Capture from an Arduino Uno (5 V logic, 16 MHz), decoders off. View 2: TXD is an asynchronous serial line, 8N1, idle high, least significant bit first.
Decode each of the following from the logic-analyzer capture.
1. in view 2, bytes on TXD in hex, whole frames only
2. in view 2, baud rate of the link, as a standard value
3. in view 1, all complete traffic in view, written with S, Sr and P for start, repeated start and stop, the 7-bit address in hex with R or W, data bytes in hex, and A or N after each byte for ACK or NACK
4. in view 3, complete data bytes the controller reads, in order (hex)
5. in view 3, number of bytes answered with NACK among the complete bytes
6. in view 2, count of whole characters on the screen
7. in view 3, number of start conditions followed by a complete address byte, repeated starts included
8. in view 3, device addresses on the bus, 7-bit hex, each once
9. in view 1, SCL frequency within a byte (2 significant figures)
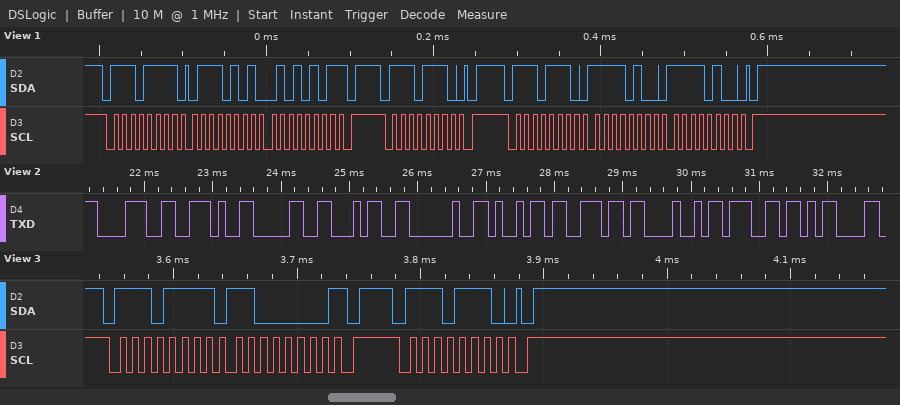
38 2E 30 34 20 69 6E 48 67 0D
9600 baud
S 77R A 75 A 55 N P S 77W A P S 77W A F4 A F4 A P
C0
1
10
2
0x77
100 kHz
